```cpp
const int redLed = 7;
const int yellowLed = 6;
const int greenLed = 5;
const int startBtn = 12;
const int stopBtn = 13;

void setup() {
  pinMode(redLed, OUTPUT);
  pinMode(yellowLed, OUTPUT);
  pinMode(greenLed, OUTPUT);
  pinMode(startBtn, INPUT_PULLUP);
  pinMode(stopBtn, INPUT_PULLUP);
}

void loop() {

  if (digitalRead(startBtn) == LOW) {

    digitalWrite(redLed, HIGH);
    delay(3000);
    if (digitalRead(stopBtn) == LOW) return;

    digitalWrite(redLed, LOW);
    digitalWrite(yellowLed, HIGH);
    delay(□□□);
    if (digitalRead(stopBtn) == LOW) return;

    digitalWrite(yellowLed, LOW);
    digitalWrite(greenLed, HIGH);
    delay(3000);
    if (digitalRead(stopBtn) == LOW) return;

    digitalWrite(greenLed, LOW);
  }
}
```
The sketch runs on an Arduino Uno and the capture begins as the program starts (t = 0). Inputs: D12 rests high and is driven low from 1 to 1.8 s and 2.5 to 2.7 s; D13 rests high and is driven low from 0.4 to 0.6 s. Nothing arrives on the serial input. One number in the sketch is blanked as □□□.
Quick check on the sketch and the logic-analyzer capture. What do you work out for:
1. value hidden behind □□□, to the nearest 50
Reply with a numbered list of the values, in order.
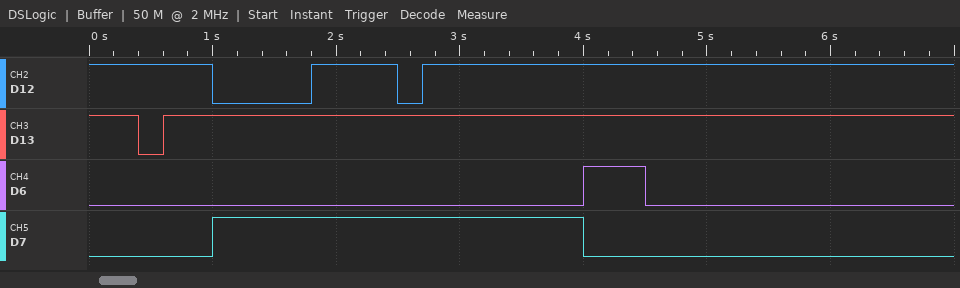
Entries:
1. 500
